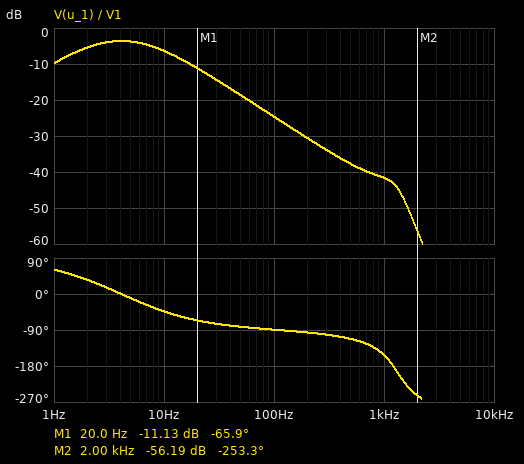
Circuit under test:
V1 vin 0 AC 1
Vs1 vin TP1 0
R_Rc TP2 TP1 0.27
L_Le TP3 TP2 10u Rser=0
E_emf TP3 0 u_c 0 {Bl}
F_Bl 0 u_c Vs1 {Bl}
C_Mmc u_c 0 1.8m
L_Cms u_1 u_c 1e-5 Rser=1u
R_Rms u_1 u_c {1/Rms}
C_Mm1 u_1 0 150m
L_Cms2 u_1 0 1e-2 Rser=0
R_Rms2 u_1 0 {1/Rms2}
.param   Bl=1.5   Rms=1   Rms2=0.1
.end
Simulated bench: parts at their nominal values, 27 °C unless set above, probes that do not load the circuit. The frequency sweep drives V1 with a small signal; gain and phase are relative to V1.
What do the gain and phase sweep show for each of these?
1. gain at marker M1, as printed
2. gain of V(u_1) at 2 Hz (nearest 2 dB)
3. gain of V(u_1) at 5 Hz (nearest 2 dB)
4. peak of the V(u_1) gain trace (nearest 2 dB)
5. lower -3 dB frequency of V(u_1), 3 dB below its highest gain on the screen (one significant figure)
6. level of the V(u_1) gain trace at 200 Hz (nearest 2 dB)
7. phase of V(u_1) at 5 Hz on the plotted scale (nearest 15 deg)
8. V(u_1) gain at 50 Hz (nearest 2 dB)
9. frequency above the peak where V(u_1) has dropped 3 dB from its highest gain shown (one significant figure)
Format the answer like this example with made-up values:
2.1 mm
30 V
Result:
-11.13 dB
-6 dB
-4 dB
-4 dB
2 Hz
-30 dB
-15 deg
-18 dB
10 Hz
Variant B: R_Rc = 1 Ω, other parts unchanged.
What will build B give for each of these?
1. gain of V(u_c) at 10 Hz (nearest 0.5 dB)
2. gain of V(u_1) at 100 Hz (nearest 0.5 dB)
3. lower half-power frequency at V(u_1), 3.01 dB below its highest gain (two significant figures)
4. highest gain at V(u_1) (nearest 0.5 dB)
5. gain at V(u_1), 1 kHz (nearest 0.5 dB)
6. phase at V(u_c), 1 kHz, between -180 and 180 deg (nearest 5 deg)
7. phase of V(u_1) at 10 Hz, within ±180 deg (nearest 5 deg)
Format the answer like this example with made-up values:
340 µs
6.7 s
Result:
-15.0 dB
-36.0 dB
3.0 Hz
-4.0 dB
-47.5 dB
55 deg
-75 deg
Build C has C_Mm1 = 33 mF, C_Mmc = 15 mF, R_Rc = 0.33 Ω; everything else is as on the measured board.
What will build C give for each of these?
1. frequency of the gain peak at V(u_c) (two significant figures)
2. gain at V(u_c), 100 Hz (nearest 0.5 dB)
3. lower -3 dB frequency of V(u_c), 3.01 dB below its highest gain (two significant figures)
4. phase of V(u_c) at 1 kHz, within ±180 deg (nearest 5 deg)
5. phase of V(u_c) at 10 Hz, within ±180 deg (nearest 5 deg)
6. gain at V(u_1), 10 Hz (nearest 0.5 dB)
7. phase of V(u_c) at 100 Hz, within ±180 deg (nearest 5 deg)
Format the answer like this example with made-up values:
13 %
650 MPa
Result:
7.3 Hz
-17.5 dB
2.1 Hz
-95 deg
-10 deg
-4.0 dB
-80 deg
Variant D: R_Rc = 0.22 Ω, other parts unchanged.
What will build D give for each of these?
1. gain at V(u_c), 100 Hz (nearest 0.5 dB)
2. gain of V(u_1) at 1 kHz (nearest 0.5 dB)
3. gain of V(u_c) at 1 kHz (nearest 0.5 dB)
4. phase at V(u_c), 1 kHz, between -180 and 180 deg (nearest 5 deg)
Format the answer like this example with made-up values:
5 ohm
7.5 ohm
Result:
-30.5 dB
-41.0 dB
-6.0 dB
20 deg
